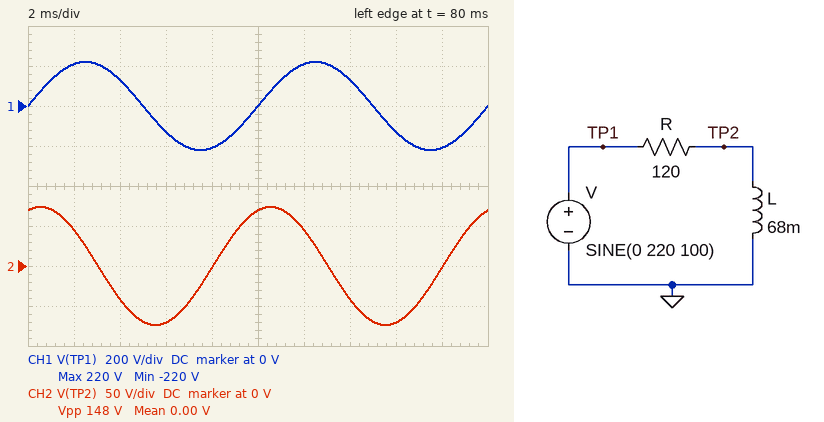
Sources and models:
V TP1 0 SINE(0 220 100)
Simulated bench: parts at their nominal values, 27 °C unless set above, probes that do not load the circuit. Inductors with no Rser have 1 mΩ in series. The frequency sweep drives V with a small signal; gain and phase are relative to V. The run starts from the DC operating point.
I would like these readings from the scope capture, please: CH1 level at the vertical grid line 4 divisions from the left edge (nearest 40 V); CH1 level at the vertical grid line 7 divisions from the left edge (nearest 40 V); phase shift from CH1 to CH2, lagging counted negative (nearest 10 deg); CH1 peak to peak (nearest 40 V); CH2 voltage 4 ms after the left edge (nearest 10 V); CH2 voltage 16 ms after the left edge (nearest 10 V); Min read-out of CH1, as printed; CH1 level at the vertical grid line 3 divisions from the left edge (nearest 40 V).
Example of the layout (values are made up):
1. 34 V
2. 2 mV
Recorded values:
1. -200 V
2. 120 V
3. 70 deg
4. 440 V
5. -40 V
6. -70 V
7. -220 V
8. -120 V
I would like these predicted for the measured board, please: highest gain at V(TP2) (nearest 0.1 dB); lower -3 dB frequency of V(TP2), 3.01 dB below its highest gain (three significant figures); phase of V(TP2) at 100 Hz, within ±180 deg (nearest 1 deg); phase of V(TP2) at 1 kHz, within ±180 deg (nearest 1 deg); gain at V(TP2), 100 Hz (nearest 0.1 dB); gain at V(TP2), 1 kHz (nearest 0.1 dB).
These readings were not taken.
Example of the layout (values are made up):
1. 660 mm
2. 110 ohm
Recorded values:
1. 0 dB
2. 281 Hz
3. 70 deg
4. 16 deg
5. -9.5 dB
6. -0.3 dB
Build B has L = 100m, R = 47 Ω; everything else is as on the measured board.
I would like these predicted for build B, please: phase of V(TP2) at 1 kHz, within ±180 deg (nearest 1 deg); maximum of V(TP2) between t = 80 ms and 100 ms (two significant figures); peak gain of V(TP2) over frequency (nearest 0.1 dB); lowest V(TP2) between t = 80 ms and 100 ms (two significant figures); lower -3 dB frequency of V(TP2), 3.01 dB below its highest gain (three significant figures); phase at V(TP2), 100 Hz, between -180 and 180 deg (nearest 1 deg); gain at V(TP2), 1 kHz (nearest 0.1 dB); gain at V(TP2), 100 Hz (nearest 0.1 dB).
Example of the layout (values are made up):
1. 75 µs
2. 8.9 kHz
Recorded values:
1. 4 deg
2. 180 V
3. 0 dB
4. -180 V
5. 74.8 Hz
6. 37 deg
7. 0 dB
8. -1.9 dB
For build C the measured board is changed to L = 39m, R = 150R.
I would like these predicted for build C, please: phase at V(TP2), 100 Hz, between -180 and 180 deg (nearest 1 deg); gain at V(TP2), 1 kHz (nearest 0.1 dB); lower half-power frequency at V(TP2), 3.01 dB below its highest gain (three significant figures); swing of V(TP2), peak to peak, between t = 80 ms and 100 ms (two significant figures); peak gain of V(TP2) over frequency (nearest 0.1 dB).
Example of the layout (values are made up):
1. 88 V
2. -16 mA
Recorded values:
1. 81 deg
2. -1.4 dB
3. 612 Hz
4. 71 V
5. 0 dB
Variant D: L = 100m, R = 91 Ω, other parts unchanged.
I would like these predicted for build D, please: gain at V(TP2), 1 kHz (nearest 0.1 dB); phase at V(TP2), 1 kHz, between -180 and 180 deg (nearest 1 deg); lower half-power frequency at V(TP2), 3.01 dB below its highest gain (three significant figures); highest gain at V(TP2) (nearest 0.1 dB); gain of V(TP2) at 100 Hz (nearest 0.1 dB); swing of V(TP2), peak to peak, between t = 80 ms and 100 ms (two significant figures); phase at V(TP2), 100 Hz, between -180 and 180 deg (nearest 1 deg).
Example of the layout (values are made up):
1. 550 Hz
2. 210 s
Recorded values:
1. -0.1 dB
2. 8 deg
3. 145 Hz
4. 0 dB
5. -4.9 dB
6. 250 V
7. 55 deg
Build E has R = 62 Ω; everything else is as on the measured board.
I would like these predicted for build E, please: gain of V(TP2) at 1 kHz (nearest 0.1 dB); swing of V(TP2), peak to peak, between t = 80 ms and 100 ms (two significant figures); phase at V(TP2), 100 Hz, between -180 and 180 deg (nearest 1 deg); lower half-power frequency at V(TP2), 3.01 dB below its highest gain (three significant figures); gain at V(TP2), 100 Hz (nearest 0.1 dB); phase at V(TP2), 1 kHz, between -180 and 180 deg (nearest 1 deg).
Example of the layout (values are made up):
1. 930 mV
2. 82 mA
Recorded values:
1. -0.1 dB
2. 250 V
3. 55 deg
4. 145 Hz
5. -4.9 dB
6. 8 deg
